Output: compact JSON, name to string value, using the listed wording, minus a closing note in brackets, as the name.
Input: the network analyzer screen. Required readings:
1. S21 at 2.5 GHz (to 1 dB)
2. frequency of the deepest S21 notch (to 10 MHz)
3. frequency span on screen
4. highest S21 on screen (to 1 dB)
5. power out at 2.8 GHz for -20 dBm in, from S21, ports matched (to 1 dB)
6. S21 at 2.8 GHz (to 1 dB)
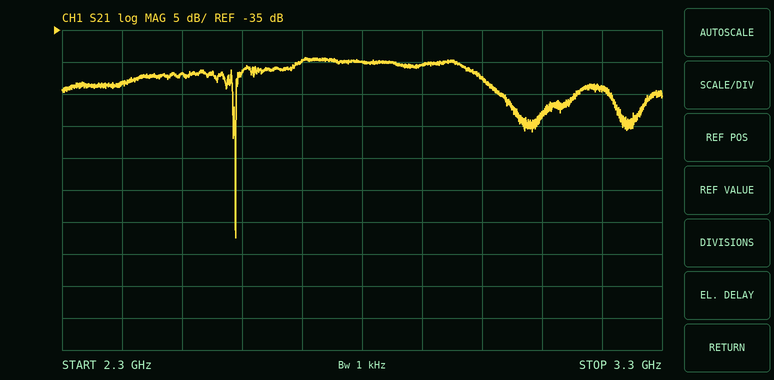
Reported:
{"S21 at 2.5 GHz": "-42 dB", "frequency of the deepest S21 notch": "2.59 GHz", "frequency span on screen": "1 GHz", "highest S21 on screen": "-39 dB", "power out at 2.8 GHz for -20 dBm in, from S21, ports matched": "-60 dBm", "S21 at 2.8 GHz": "-40 dB"}
